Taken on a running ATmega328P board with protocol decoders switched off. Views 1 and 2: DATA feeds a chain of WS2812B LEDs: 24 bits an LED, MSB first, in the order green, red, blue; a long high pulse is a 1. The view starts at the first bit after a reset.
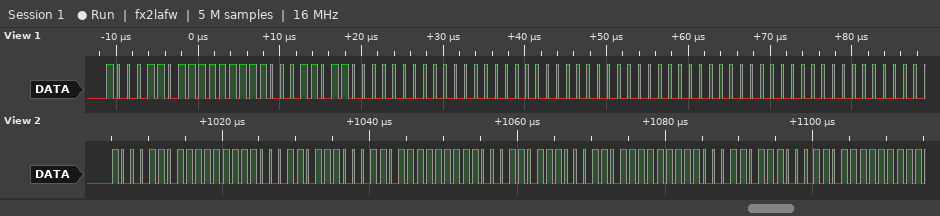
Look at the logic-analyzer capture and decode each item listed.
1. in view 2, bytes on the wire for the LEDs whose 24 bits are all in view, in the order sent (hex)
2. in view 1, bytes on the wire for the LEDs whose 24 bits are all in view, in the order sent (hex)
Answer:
8D FF 1B 8D FF 1B 8D FF 1B
8D FF 1B 00 00 00 00 00 00
